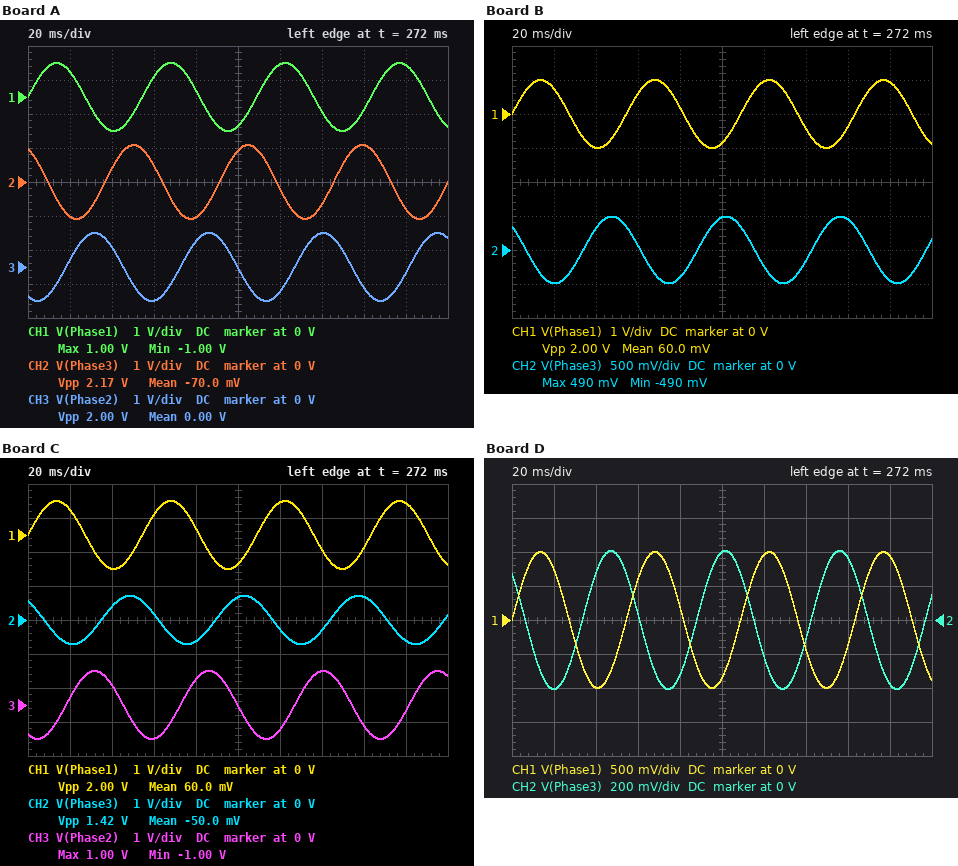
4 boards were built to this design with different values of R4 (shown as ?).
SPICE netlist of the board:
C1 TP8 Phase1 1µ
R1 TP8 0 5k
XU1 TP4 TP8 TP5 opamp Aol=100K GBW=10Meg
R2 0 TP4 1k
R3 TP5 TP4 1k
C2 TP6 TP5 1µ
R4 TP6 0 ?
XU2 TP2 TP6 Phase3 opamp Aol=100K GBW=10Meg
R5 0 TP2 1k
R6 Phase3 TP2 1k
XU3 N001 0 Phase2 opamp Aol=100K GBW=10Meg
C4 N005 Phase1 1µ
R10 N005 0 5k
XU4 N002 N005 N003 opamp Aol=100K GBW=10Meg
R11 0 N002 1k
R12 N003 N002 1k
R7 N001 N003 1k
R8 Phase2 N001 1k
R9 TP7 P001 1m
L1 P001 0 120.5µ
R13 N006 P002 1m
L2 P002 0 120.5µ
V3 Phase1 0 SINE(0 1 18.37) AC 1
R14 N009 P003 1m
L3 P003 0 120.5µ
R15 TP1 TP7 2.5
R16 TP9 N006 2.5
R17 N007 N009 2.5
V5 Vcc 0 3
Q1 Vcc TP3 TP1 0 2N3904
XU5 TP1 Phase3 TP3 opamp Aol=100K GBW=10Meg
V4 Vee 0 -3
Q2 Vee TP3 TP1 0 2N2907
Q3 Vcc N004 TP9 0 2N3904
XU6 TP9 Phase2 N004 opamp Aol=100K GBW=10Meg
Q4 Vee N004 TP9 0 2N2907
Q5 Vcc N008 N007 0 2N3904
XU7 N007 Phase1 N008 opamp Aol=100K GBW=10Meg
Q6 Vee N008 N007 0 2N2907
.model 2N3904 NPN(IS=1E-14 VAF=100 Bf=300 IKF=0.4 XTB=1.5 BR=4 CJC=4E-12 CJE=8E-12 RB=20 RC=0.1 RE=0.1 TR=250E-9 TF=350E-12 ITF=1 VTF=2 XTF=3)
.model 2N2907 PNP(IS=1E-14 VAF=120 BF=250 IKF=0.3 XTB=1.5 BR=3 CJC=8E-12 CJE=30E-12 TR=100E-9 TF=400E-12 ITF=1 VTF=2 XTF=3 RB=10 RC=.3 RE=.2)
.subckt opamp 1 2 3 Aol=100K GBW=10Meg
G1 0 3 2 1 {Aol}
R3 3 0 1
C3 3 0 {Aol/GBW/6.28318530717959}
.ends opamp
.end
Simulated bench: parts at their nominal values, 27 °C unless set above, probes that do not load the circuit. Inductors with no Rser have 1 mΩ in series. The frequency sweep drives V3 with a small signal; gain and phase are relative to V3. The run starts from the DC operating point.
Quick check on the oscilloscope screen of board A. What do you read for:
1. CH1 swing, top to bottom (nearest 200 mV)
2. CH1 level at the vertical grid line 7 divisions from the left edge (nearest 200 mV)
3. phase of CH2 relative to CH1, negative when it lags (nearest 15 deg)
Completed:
2.0 V
-400 mV
120 deg
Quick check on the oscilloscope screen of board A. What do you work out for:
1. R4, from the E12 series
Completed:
5.6 kΩ
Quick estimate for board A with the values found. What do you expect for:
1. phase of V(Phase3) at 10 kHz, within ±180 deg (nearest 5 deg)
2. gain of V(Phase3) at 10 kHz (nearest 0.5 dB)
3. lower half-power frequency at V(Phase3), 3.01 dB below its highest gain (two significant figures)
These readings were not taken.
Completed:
0 deg
12.0 dB
47 Hz
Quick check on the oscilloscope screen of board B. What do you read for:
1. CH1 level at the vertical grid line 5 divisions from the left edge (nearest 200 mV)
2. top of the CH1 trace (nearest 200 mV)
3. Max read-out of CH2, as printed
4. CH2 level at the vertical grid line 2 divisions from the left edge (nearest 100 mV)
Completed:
-800 mV
1.0 V
490 mV
300 mV
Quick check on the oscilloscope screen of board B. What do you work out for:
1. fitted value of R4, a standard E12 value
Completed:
2.2 kΩ
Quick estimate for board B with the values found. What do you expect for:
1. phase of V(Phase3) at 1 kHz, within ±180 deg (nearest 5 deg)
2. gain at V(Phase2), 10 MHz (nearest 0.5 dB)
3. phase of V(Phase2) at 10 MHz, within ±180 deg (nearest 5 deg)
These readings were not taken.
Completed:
5 deg
-8.0 dB
55 deg
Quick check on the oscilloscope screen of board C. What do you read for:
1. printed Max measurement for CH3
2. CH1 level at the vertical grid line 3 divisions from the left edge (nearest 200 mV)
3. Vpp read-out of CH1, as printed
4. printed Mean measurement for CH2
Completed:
1.00 V
600 mV
2.00 V
-50.0 mV
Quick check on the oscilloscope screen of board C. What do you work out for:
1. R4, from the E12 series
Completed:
3.3 kΩ
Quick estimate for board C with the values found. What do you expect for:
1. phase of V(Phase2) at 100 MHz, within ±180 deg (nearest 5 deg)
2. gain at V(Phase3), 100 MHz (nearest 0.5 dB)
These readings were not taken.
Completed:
5 deg
-40.0 dB
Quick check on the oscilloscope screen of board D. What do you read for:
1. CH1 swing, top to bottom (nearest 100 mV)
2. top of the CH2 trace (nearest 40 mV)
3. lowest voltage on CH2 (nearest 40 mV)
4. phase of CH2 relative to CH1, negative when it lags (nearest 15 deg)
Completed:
2.0 V
400 mV
-400 mV
135 deg
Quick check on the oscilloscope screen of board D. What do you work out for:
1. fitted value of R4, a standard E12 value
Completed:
1.8 kΩ
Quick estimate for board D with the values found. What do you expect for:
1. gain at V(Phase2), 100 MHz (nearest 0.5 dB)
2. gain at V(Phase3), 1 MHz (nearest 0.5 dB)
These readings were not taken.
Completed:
-46.0 dB
11.5 dB
